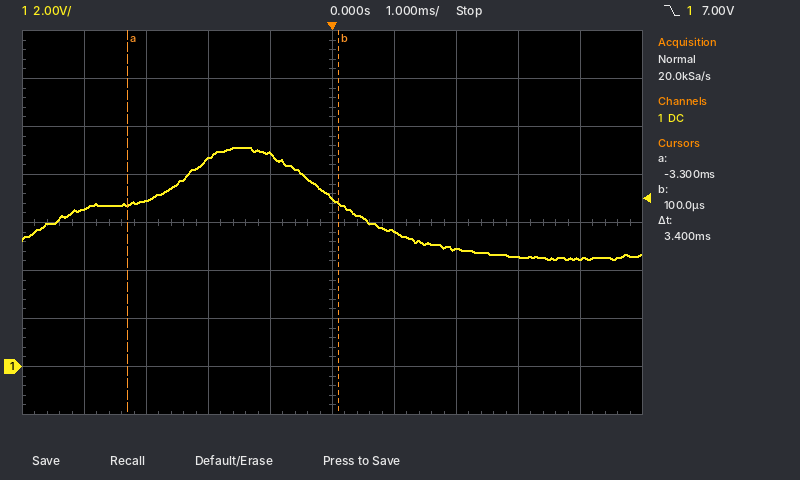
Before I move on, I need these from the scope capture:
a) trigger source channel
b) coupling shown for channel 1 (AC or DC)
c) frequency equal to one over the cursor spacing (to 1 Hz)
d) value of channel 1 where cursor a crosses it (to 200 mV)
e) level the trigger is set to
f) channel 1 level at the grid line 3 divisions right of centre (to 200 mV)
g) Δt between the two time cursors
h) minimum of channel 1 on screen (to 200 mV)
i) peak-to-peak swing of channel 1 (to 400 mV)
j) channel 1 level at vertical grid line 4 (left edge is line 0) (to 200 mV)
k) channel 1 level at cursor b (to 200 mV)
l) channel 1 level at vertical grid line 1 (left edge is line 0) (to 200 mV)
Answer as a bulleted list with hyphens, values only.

- channel 1
- DC
- 294 Hz
- 6.8 V
- 7.00 V
- 4.6 V
- 3.4 ms
- 4.4 V
- 4.8 V
- 8.8 V
- 6.8 V
- 6.6 V
